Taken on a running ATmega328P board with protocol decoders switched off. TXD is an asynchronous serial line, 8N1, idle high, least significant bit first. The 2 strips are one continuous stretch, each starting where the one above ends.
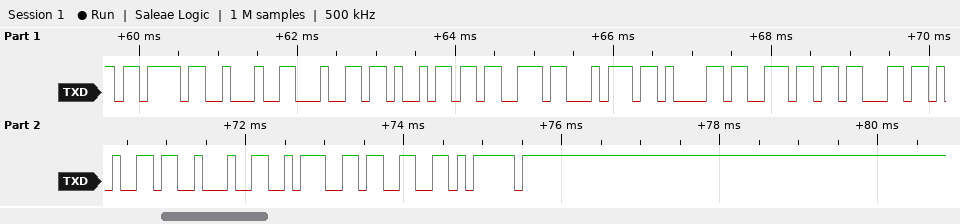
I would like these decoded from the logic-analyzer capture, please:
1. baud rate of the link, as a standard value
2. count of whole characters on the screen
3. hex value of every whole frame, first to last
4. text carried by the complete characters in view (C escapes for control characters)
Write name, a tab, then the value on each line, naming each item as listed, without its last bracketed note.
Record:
baud rate of the link, as a standard value	9600 baud
count of whole characters on the screen	14
hex value of every whole frame, first to last	0x7B 0x22 0x64 0x69 0x73 0x74 0x61 0x6E 0x63 0x65 0x22 0x3A 0x33 0x7D
text carried by the complete characters in view	"{\"distance\":3}"
